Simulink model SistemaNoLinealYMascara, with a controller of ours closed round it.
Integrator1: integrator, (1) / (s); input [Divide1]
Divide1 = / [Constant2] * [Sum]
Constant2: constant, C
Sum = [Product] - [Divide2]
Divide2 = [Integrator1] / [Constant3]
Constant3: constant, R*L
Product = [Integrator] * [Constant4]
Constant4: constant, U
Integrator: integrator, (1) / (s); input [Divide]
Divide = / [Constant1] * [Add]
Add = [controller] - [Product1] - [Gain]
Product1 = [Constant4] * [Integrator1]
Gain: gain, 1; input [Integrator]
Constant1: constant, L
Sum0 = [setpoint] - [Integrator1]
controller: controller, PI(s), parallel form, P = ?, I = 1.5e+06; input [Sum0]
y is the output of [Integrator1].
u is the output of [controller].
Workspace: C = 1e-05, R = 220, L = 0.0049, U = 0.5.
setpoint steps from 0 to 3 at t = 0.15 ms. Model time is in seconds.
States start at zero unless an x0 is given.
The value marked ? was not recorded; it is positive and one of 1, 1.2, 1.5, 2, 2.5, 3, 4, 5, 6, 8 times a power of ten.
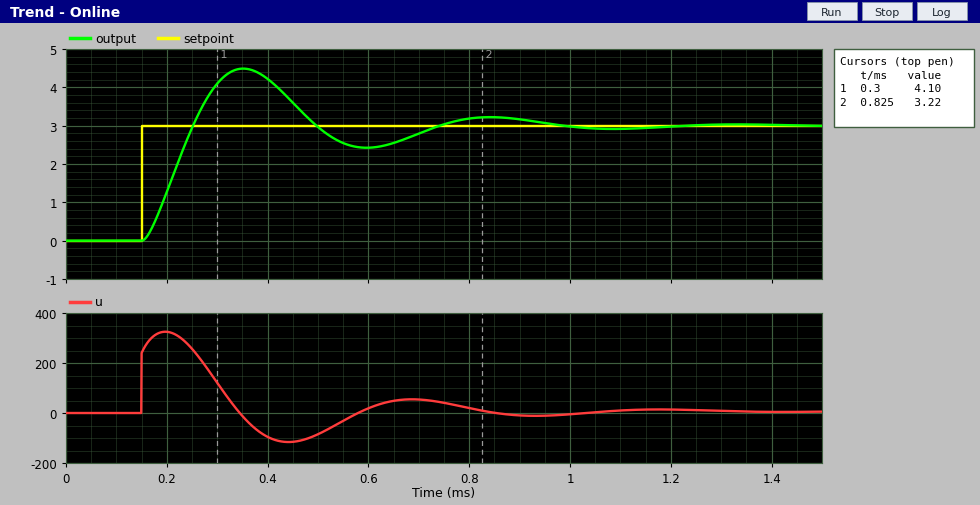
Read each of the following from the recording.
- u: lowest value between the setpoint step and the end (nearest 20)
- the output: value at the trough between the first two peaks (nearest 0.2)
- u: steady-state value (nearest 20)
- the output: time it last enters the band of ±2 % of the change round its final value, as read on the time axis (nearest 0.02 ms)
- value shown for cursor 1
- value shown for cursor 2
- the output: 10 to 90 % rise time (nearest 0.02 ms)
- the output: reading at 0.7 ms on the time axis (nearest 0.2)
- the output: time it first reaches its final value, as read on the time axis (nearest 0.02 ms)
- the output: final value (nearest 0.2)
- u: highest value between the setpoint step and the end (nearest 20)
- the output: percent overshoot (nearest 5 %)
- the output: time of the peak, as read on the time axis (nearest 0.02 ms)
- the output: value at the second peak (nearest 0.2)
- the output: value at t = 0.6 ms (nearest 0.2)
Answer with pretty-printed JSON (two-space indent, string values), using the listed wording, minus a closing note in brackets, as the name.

{
  "u: lowest value between the setpoint step and the end": "-120",
  "the output: value at the trough between the first two peaks": "2.4",
  "u: steady-state value": "0",
  "the output: time it last enters the band of ±2 % of the change round its final value, as read on the time axis": "1.16 ms",
  "value shown for cursor 1": "4.10",
  "value shown for cursor 2": "3.22",
  "the output: 10 to 90 % rise time": "0.08 ms",
  "the output: reading at 0.7 ms on the time axis": "2.8",
  "the output: time it first reaches its final value, as read on the time axis": "0.26 ms",
  "the output: final value": "3.0",
  "u: highest value between the setpoint step and the end": "320",
  "the output: percent overshoot": "50 %",
  "the output: time of the peak, as read on the time axis": "0.36 ms",
  "the output: value at the second peak": "3.2",
  "the output: value at t = 0.6 ms": "2.4"
}
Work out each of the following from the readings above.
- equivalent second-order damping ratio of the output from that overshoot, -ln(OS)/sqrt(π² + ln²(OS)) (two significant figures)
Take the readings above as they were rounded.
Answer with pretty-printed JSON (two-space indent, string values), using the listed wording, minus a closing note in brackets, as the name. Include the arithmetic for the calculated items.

{
  "equivalent second-order damping ratio of the output from that overshoot, -ln(OS)/sqrt(π² + ln²(OS))": "ln(0.5) = -0.693; 0.693 / sqrt(9.870 + 0.480) = 0.22"
}
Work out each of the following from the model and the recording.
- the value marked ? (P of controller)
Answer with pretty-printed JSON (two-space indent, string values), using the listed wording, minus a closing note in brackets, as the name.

{
  "the value marked ?": "80"
}
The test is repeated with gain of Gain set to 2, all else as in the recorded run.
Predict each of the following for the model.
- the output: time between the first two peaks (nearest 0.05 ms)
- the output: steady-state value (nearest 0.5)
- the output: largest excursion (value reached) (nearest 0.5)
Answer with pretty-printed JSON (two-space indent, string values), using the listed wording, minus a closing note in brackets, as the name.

{
  "the output: time between the first two peaks": "0.50 ms",
  "the output: steady-state value": "3.0",
  "the output: largest excursion (value reached)": "4.5"
}
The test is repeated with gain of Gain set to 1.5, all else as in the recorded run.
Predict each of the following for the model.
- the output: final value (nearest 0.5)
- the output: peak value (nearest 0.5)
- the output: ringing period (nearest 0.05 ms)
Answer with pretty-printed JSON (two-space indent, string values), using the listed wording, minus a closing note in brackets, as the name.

{
  "the output: final value": "3.0",
  "the output: peak value": "4.5",
  "the output: ringing period": "0.50 ms"
}
